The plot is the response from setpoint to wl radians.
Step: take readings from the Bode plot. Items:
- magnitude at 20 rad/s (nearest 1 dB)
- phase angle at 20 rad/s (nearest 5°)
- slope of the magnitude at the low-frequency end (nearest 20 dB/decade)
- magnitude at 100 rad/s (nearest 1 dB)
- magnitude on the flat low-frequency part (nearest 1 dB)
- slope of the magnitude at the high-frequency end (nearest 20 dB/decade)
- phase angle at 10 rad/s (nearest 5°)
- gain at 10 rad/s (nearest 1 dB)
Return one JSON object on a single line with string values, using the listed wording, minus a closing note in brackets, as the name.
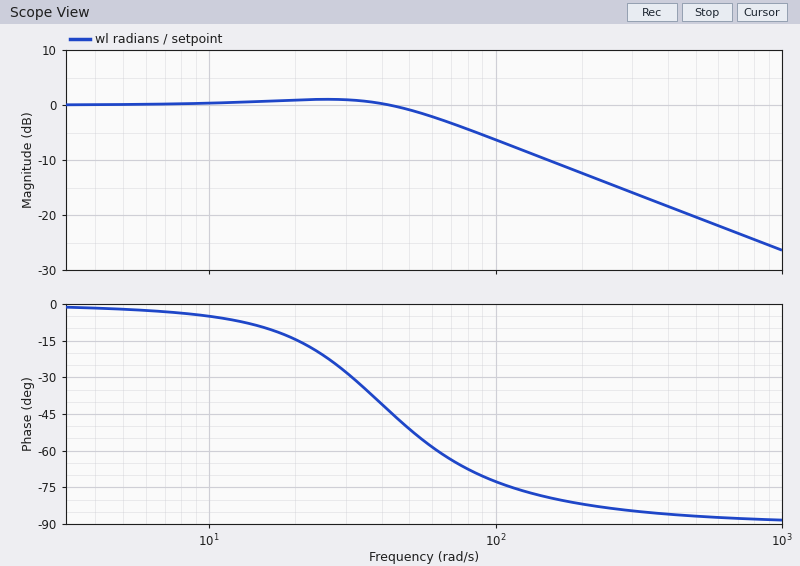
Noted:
{"magnitude at 20 rad/s": "1 dB", "phase angle at 20 rad/s": "-15°", "slope of the magnitude at the low-frequency end": "0 dB/decade", "magnitude at 100 rad/s": "-6 dB", "magnitude on the flat low-frequency part": "0 dB", "slope of the magnitude at the high-frequency end": "-20 dB/decade", "phase angle at 10 rad/s": "-5°", "gain at 10 rad/s": "0 dB"}
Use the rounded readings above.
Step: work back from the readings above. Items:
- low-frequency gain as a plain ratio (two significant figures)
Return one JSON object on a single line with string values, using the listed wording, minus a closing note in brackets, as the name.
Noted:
{"low-frequency gain as a plain ratio": "1.0"}
